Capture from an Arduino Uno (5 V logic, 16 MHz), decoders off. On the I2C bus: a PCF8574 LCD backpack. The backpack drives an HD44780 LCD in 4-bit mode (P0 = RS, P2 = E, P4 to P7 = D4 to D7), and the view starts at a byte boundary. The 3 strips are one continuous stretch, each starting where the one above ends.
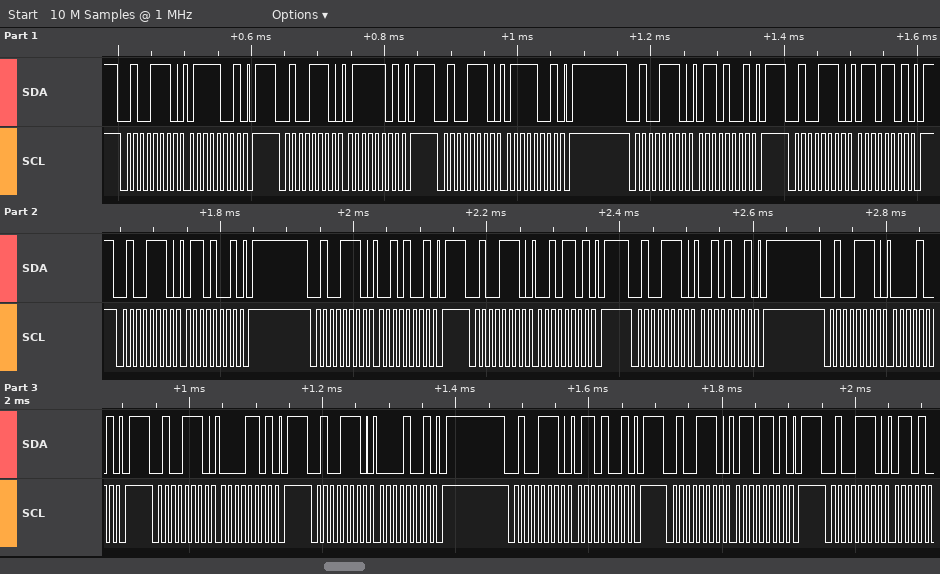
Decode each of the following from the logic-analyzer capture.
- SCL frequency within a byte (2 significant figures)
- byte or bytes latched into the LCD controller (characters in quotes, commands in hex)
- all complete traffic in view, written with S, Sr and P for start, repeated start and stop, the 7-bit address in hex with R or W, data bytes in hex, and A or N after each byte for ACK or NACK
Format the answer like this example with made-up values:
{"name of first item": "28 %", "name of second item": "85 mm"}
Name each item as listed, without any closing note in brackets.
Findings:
{"SCL frequency within a byte": "100 kHz", "byte or bytes latched into the LCD controller": "'v' ' '", "all complete traffic in view, written with S, Sr and P for start, repeated start and stop, the 7-bit address in hex with R or W, data bytes in hex, and A or N after each byte for ACK or NACK": "S 27W A 79 A P S 27W A 7D A P S 27W A 79 A P S 27W A 69 A P S 27W A 6D A P S 27W A 69 A P S 27W A 29 A P S 27W A 2D A P S 27W A 29 A P S 27W A 09 A P S 27W A 0D A P S 27W A 09 A P S 27W A 69 A P S 27W A 6D A P S 27W A"}
